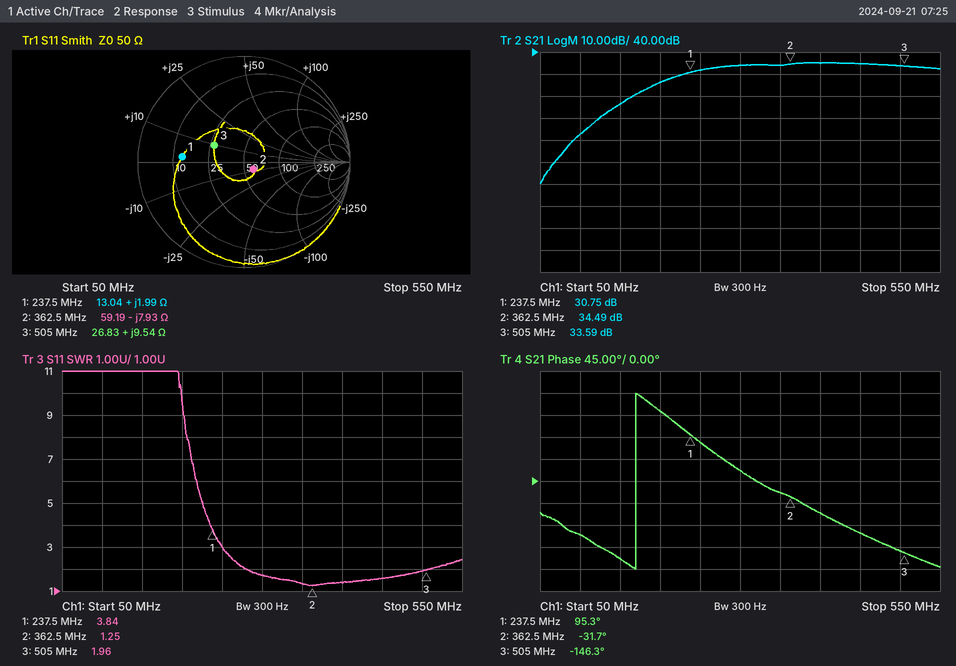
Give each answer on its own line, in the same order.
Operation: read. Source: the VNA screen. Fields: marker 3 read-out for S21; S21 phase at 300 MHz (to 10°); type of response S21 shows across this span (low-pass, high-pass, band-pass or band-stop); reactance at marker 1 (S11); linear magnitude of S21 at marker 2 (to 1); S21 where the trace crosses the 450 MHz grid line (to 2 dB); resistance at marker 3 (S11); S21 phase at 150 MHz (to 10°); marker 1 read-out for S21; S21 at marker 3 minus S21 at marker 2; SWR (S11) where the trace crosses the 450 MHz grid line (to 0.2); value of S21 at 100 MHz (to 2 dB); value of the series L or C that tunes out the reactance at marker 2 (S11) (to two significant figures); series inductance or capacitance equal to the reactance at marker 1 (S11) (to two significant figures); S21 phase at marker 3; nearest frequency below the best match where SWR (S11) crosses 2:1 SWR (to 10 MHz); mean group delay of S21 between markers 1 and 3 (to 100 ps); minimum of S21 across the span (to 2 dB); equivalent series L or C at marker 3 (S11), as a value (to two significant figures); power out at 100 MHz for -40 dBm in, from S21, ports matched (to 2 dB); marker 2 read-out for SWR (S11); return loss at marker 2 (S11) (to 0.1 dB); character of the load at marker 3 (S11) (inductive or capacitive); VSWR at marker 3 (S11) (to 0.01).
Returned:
33.59 dB
20°
high-pass
+1.99 Ω
53
34 dB
26.83 Ω
-160°
30.75 dB
-0.90 dB
1.6
2 dB
3.5 nH
1.3 nH
-146.3°
280 MHz
2.5 ns
-20 dB
3.0 nH
-38 dBm
1.25
19.1 dB
inductive
1.96
